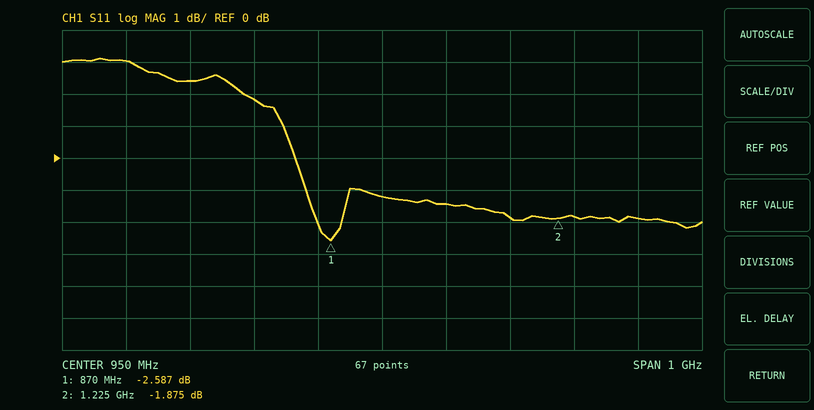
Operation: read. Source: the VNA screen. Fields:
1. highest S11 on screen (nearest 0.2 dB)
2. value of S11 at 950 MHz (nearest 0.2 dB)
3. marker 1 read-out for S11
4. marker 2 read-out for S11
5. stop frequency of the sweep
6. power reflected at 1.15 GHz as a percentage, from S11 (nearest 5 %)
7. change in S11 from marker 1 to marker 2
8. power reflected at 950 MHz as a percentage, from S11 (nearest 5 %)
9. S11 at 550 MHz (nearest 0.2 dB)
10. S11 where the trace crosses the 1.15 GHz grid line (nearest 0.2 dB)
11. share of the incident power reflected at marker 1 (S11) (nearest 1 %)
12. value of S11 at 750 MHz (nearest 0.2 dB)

3.2 dB
-1.2 dB
-2.587 dB
-1.875 dB
1.45 GHz
65 %
0.712 dB
75 %
3.0 dB
-1.8 dB
55 %
1.8 dB
